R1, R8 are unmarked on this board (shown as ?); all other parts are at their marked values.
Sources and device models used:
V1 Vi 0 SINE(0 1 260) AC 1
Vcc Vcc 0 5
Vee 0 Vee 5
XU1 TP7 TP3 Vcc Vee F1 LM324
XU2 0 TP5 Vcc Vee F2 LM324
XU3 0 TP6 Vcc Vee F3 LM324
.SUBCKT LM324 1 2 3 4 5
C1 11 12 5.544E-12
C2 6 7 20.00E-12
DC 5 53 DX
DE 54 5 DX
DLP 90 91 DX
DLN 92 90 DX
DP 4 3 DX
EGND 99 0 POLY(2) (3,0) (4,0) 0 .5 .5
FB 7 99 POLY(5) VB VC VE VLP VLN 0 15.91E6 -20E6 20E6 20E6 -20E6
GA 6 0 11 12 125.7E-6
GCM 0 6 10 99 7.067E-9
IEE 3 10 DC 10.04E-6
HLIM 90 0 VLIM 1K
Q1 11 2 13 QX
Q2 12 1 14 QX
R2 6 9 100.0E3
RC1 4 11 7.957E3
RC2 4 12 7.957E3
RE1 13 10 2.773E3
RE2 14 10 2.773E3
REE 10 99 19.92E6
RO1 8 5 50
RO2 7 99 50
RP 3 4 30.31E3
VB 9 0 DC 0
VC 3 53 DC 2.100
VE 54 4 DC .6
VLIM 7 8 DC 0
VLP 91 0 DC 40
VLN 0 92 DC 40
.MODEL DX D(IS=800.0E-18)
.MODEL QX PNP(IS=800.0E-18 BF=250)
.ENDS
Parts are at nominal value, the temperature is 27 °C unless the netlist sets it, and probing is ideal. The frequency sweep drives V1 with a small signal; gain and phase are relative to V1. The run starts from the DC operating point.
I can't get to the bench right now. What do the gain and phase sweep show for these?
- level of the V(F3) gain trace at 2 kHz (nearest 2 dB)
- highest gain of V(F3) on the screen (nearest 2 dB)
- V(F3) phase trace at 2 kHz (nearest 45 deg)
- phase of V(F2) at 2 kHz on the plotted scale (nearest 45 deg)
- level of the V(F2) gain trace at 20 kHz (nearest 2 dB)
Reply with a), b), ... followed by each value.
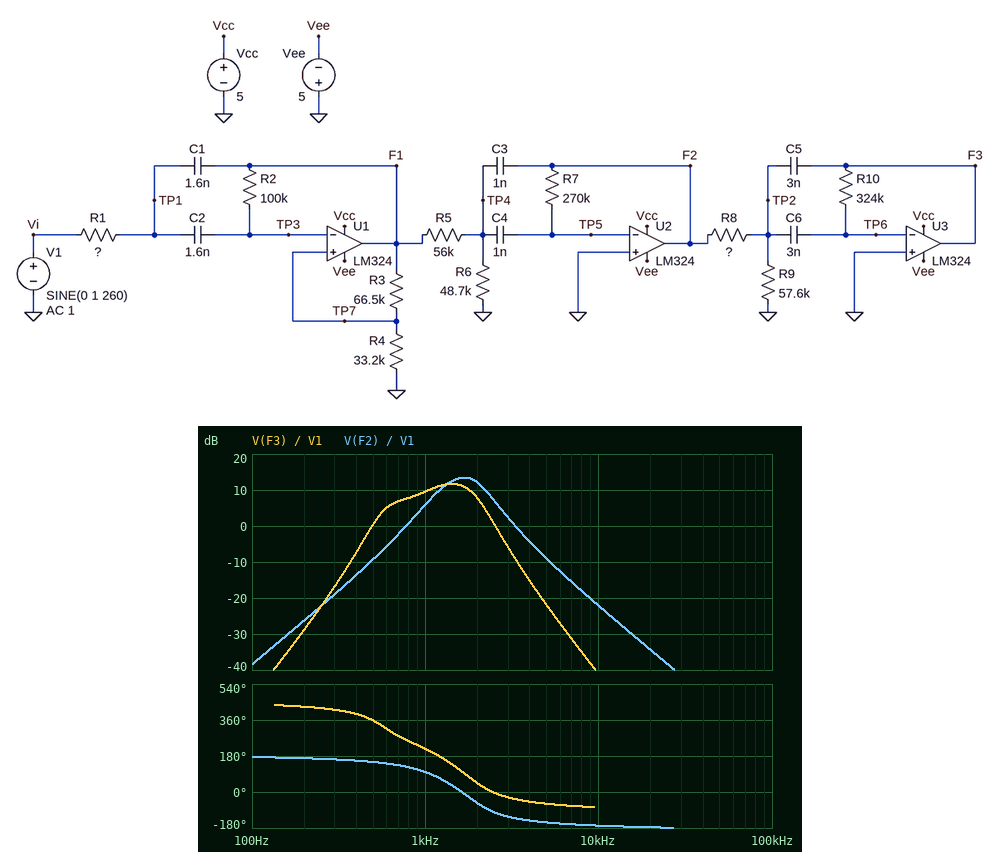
a) 8 dB
b) 12 dB
c) 45 deg
d) -45 deg
e) -34 dB
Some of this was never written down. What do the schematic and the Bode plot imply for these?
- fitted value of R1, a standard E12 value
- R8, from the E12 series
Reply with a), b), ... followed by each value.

a) 56 kΩ
b) 47 kΩ
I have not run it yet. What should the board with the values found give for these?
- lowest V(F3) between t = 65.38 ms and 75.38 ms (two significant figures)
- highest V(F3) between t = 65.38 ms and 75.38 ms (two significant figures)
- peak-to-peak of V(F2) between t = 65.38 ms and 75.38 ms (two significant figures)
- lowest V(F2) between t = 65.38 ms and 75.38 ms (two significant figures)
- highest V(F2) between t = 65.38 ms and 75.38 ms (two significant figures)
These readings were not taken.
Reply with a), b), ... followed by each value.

a) -94 mV
b) 81 mV
c) 170 mV
d) -89 mV
e) 78 mV
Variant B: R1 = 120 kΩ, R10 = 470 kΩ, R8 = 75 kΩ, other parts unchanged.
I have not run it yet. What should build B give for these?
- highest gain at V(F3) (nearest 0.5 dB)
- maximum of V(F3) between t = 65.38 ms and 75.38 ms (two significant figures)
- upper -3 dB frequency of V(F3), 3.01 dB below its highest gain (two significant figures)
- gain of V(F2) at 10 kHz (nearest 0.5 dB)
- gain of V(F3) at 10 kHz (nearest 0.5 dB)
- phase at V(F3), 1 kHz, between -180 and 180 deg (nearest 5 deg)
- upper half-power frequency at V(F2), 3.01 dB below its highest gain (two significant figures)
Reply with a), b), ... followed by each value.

a) -3.0 dB
b) 100 mV
c) 2.0 kHz
d) -29.0 dB
e) -52.0 dB
f) 165 deg
g) 2.3 kHz
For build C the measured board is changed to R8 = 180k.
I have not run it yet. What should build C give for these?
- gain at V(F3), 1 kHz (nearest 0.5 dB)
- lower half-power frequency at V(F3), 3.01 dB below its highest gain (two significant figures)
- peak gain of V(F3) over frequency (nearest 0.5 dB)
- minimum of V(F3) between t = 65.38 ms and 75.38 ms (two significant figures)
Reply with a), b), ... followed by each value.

a) -3.5 dB
b) 990 Hz
c) -0.5 dB
d) -47 mV
